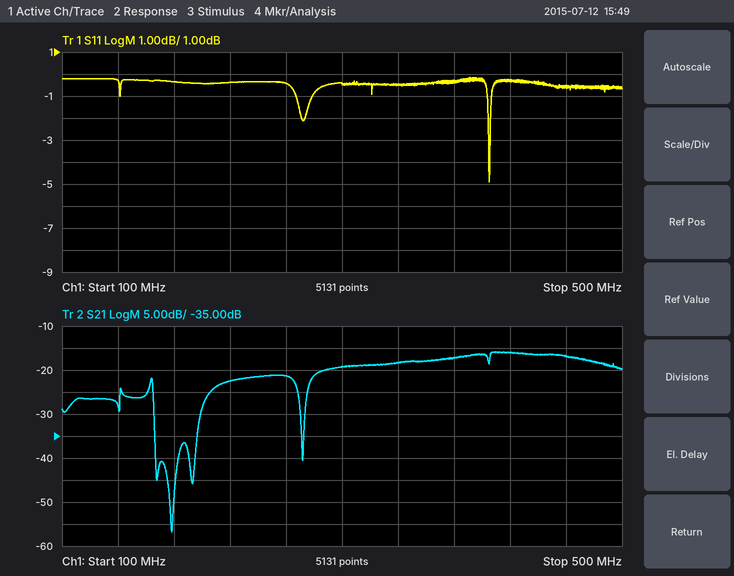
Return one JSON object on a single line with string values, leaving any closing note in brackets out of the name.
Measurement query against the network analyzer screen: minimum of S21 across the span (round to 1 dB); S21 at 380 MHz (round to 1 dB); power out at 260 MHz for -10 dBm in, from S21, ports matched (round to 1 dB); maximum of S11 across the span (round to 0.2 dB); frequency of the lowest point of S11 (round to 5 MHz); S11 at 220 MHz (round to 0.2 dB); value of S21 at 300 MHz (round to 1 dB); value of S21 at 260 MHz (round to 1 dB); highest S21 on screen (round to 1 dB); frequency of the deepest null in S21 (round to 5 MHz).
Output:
{"minimum of S21 across the span": "-57 dB", "S21 at 380 MHz": "-17 dB", "power out at 260 MHz for -10 dBm in, from S21, ports matched": "-31 dBm", "maximum of S11 across the span": "-0.2 dB", "frequency of the lowest point of S11": "405 MHz", "S11 at 220 MHz": "-0.4 dB", "value of S21 at 300 MHz": "-19 dB", "value of S21 at 260 MHz": "-21 dB", "highest S21 on screen": "-16 dB", "frequency of the deepest null in S21": "180 MHz"}
